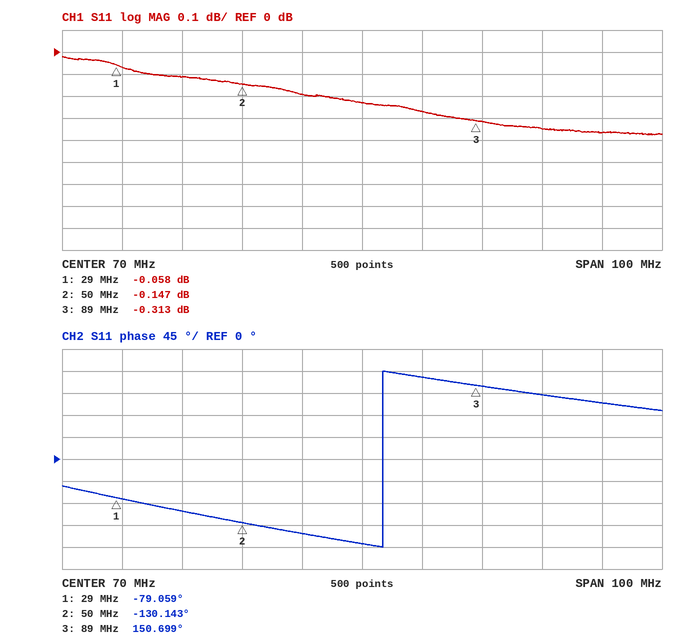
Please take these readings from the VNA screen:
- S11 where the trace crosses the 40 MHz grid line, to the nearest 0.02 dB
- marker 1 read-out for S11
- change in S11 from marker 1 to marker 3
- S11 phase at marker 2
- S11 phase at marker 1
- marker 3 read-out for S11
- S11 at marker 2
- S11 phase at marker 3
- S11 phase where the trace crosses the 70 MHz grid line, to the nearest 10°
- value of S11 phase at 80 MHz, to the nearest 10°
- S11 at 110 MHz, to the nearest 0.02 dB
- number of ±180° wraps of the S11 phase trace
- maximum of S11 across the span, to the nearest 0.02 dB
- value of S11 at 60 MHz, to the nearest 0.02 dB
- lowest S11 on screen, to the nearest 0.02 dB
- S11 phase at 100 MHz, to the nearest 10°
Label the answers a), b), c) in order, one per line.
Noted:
a) -0.12 dB
b) -0.058 dB
c) -0.255 dB
d) -130.143°
e) -79.059°
f) -0.313 dB
g) -0.147 dB
h) 150.699°
i) -170°
j) 170°
k) -0.36 dB
l) 1
m) -0.02 dB
n) -0.20 dB
o) -0.38 dB
p) 130°
